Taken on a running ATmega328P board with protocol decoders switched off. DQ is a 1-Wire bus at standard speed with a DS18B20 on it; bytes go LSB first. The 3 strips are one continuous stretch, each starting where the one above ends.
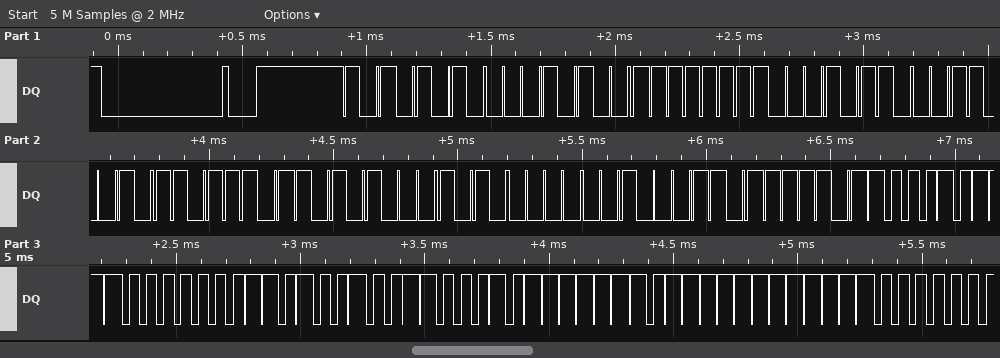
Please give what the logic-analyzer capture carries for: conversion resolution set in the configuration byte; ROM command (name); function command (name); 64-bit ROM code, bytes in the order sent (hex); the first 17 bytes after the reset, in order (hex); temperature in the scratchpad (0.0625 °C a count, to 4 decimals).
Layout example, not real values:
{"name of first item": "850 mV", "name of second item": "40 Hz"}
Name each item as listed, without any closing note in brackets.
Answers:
{"conversion resolution set in the configuration byte": "12 bits", "ROM command": "Match ROM", "function command": "Read Scratchpad", "64-bit ROM code, bytes in the order sent": "28 FF 68 4C BB 15 05 C4", "the first 17 bytes after the reset, in order": "55 28 FF 68 4C BB 15 05 C4 BE D1 01 4B 46 7F FF 0F", "temperature in the scratchpad": "29.0625 °C"}
